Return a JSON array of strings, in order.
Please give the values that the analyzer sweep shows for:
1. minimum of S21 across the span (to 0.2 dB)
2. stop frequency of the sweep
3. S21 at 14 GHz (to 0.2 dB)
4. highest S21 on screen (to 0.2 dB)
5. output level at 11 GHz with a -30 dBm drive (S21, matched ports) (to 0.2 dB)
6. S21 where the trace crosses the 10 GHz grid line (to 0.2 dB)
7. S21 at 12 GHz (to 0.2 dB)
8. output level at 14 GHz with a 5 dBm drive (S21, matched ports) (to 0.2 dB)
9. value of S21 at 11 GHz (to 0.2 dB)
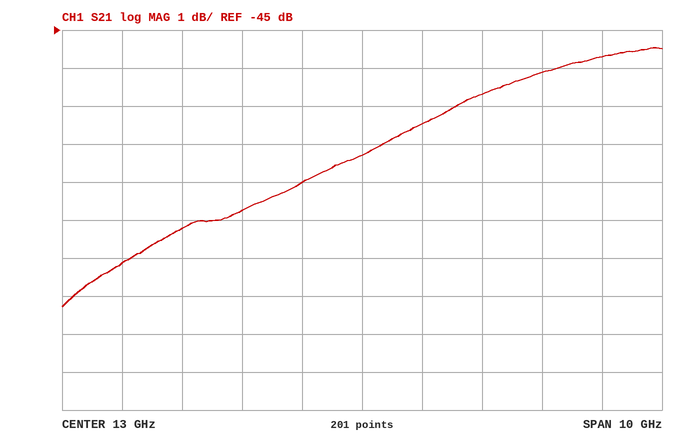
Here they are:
["-52.2 dB", "18 GHz", "-47.4 dB", "-45.4 dB", "-79.8 dBm", "-50.2 dB", "-49.0 dB", "-42.4 dBm", "-49.8 dB"]
